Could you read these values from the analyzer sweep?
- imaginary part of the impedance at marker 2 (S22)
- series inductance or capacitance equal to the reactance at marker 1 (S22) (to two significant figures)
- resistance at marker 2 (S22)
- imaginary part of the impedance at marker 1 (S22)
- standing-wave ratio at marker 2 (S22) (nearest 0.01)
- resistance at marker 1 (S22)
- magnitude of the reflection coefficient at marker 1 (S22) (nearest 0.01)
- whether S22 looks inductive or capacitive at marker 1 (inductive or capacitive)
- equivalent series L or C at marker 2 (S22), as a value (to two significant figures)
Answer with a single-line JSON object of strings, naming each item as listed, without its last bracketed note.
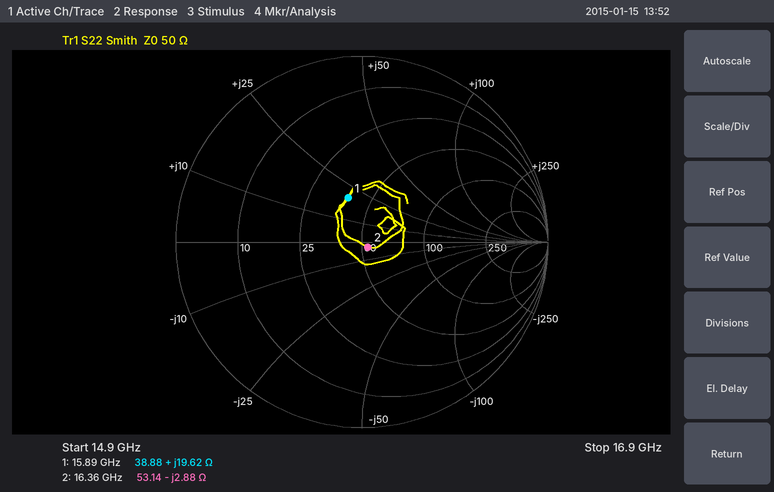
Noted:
{"imaginary part of the impedance at marker 2": "-2.88 Ω", "series inductance or capacitance equal to the reactance at marker 1 (S22)": "200 pH", "resistance at marker 2": "53.14 Ω", "imaginary part of the impedance at marker 1": "+19.62 Ω", "standing-wave ratio at marker 2 (S22)": "1.09", "resistance at marker 1": "38.88 Ω", "magnitude of the reflection coefficient at marker 1 (S22)": "0.25", "whether S22 looks inductive or capacitive at marker 1": "inductive", "equivalent series L or C at marker 2 (S22), as a value": "3.4 pF"}
